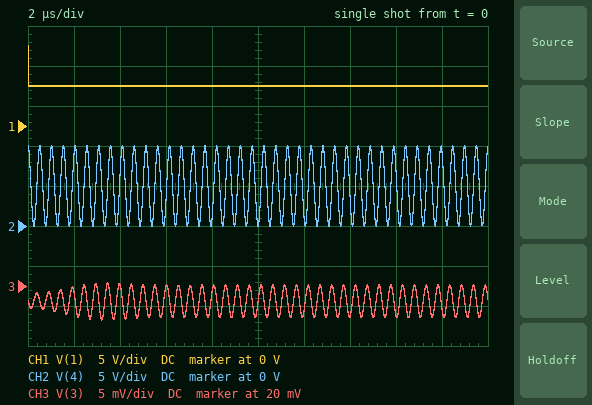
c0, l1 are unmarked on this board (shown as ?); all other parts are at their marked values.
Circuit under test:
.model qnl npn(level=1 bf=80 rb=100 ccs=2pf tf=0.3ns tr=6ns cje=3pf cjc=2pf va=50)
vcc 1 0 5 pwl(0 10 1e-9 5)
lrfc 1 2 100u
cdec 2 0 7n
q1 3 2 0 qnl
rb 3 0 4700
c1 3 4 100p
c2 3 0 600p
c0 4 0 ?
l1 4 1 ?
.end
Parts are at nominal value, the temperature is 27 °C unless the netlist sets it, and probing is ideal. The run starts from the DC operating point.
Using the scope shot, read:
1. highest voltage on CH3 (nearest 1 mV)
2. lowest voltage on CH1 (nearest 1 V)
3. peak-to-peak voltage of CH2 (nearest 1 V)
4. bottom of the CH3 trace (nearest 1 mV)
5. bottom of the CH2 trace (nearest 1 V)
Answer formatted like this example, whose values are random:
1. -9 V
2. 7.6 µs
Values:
1. 20 mV
2. 5 V
3. 10 V
4. 16 mV
5. 0 V
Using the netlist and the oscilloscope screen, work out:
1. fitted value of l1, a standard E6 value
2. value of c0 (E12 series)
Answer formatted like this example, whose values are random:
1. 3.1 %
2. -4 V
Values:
1. 10 µH
2. 560 pF
